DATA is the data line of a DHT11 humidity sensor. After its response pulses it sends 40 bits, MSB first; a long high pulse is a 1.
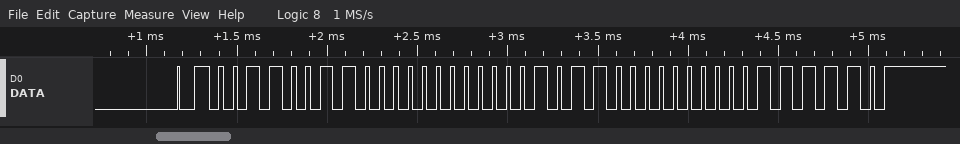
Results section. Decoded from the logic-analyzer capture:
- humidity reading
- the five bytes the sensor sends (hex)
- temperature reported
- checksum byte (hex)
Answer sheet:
51 %
33 00 0B 00 3E
11.0 °C
0x3E
